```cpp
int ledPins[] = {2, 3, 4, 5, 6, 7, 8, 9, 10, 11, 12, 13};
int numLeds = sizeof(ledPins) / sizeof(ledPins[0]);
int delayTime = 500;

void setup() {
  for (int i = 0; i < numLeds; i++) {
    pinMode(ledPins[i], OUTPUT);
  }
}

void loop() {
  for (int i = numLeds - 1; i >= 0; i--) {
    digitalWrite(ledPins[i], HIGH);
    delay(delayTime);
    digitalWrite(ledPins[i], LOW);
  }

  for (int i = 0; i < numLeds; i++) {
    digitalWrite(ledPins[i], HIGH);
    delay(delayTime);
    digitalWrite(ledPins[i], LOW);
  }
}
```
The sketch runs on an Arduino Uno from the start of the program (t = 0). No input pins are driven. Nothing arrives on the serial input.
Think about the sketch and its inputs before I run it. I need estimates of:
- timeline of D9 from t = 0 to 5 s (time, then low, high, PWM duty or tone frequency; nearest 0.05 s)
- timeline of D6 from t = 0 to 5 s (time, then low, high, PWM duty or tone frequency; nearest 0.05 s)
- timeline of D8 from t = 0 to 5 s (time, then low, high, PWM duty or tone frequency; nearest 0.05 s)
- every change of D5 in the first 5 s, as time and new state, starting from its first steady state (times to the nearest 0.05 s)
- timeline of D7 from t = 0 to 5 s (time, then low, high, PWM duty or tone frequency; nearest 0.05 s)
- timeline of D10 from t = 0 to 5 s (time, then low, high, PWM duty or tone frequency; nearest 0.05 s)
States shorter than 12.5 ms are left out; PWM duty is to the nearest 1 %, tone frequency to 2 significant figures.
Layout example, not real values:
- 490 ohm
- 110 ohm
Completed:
- 0 s low; 2 s high; 2.5 s low
- 0 s low; 3.5 s high; 4 s low
- 0 s low; 2.5 s high; 3 s low
- 0 s low; 4 s high; 4.5 s low
- 0 s low; 3 s high; 3.5 s low
- 0 s low; 1.5 s high; 2 s low
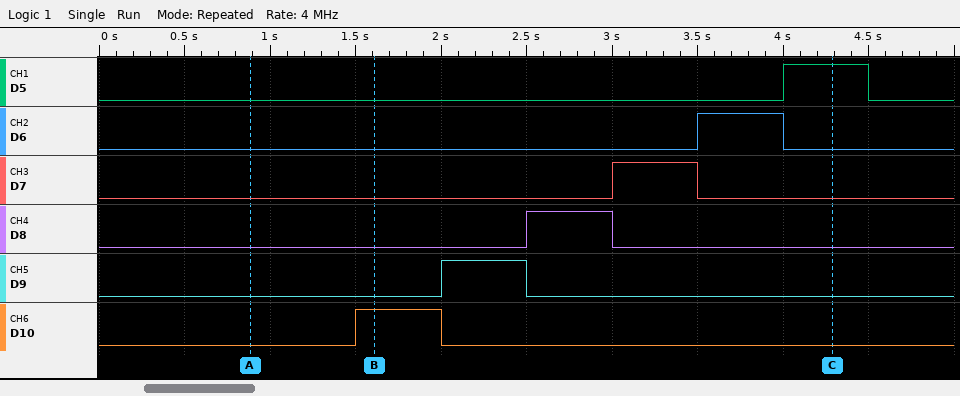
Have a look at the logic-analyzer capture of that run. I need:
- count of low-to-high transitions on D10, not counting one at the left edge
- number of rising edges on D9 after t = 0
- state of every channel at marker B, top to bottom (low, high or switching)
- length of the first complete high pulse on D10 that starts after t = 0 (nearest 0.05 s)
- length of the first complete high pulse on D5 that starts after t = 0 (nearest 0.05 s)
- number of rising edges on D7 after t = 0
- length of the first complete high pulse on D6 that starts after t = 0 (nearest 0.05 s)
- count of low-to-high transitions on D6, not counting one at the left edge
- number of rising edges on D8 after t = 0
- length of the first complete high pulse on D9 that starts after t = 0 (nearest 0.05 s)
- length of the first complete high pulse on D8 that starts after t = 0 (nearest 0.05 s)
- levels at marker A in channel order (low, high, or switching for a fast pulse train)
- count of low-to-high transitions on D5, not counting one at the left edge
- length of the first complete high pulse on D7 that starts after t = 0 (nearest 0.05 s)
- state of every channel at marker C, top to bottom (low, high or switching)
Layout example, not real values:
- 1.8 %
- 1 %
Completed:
- 1
- 1
- D5 low, D6 low, D7 low, D8 low, D9 low, D10 high
- 0.50 s
- 0.50 s
- 1
- 0.50 s
- 1
- 1
- 0.50 s
- 0.50 s
- D5 low, D6 low, D7 low, D8 low, D9 low, D10 low
- 1
- 0.50 s
- D5 high, D6 low, D7 low, D8 low, D9 low, D10 low
